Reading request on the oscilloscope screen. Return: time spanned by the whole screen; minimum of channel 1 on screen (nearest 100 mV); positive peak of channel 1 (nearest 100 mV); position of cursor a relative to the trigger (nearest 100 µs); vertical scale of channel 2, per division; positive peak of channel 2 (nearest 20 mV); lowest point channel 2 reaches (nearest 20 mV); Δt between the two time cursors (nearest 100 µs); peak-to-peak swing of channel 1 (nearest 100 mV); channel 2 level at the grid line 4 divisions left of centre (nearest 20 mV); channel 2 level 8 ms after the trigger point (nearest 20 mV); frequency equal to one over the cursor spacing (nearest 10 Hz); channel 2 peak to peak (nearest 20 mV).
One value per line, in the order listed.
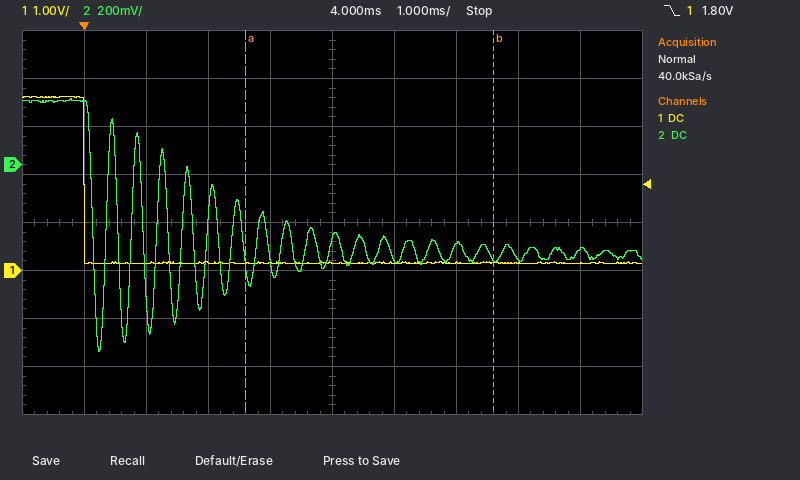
10 ms
100 mV
3.6 V
+2.6 ms
200 mV
280 mV
-780 mV
4.0 ms
3.5 V
260 mV
-360 mV
250 Hz
1.06 V
